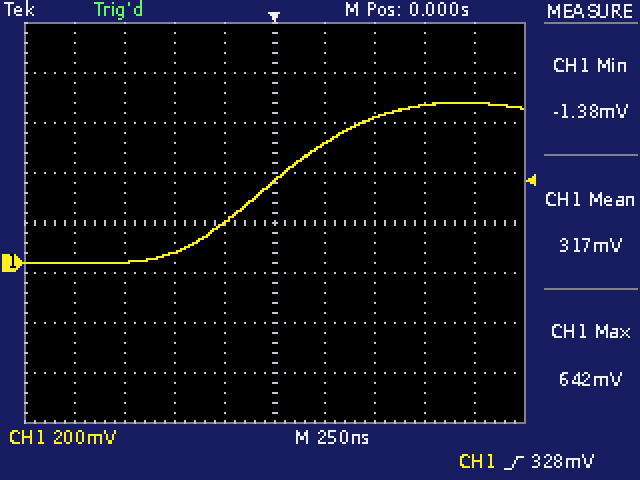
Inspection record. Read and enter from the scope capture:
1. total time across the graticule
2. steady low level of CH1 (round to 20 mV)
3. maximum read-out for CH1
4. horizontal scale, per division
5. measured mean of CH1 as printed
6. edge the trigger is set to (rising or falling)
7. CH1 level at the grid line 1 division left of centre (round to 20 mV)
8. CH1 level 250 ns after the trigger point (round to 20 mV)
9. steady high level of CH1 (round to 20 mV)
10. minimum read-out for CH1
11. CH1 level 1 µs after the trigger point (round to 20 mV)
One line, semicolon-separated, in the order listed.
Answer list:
2.5 µs; 0 mV; 642 mV; 250 ns; 317 mV; rising; 160 mV; 480 mV; 640 mV; -1.38 mV; 640 mV
